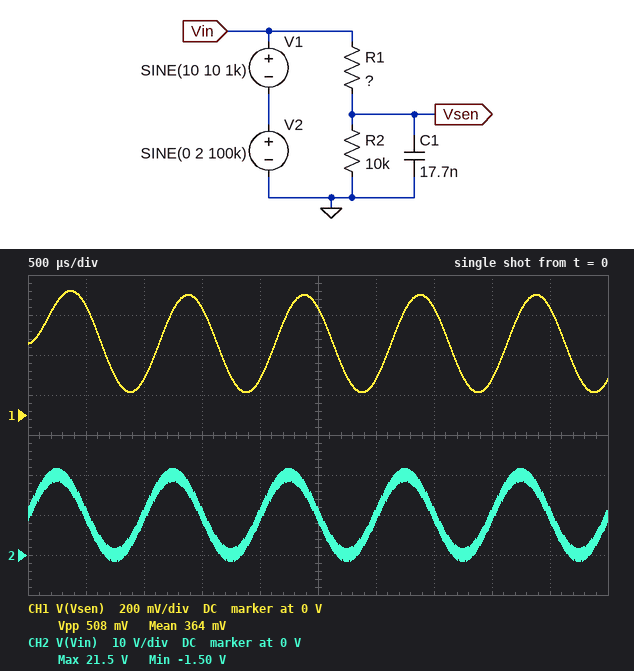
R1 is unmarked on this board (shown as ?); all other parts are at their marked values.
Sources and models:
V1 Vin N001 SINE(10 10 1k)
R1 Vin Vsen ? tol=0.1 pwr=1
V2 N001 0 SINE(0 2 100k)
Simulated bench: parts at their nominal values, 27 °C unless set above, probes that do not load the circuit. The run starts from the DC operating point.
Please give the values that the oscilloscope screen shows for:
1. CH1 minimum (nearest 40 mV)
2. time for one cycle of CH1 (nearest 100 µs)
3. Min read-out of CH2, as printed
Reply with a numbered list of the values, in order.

1. 120 mV
2. 1.0 ms
3. -1.50 V
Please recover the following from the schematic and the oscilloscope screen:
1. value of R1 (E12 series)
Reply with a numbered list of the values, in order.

1. 270 kΩ
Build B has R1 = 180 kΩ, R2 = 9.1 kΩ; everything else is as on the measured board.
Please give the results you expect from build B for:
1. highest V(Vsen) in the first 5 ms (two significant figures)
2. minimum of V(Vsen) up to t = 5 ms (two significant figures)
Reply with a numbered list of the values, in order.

1. 850 mV
2. 130 mV
